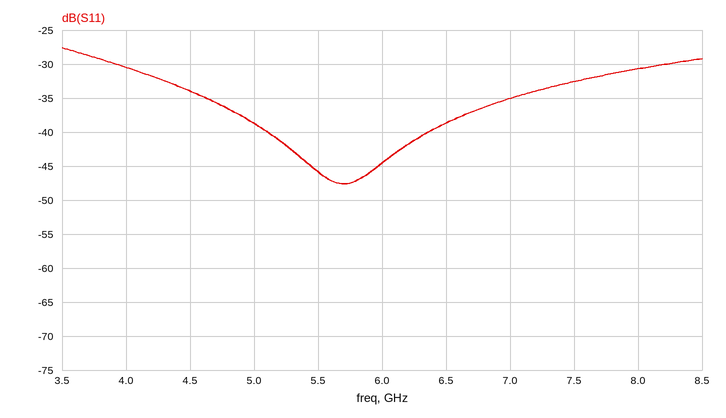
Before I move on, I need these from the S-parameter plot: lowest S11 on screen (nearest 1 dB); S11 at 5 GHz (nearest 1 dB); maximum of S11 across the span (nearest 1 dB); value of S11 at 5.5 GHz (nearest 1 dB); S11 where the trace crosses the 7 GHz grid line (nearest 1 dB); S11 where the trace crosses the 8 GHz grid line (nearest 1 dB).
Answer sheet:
-48 dB
-39 dB
-28 dB
-46 dB
-35 dB
-31 dB
